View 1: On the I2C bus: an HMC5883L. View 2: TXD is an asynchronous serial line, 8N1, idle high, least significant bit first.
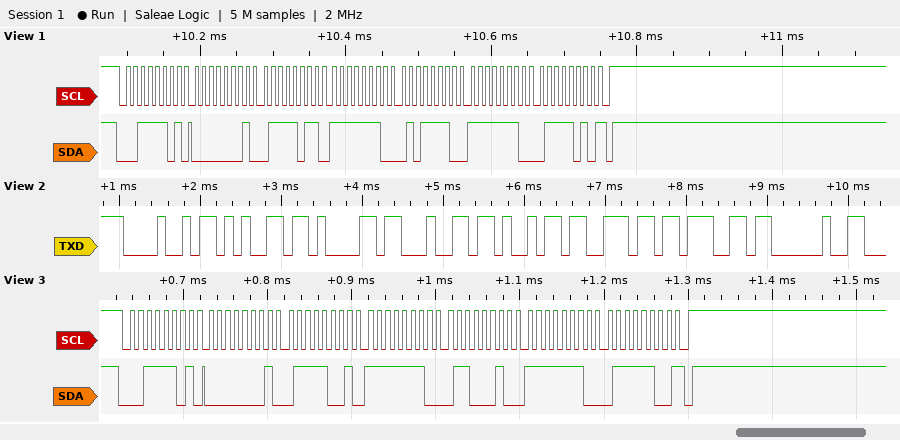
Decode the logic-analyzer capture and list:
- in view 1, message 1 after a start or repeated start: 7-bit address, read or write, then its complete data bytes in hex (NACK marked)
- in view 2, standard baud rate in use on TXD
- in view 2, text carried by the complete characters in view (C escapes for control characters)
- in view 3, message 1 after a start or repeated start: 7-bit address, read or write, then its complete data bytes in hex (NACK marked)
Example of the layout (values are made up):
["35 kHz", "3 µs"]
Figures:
["0x1E read: 01 7B FE 5E FE 7A NACK", "9600 baud", "\"Heading \"", "0x1E read: 01 79 FE 62 FE 7C NACK"]
